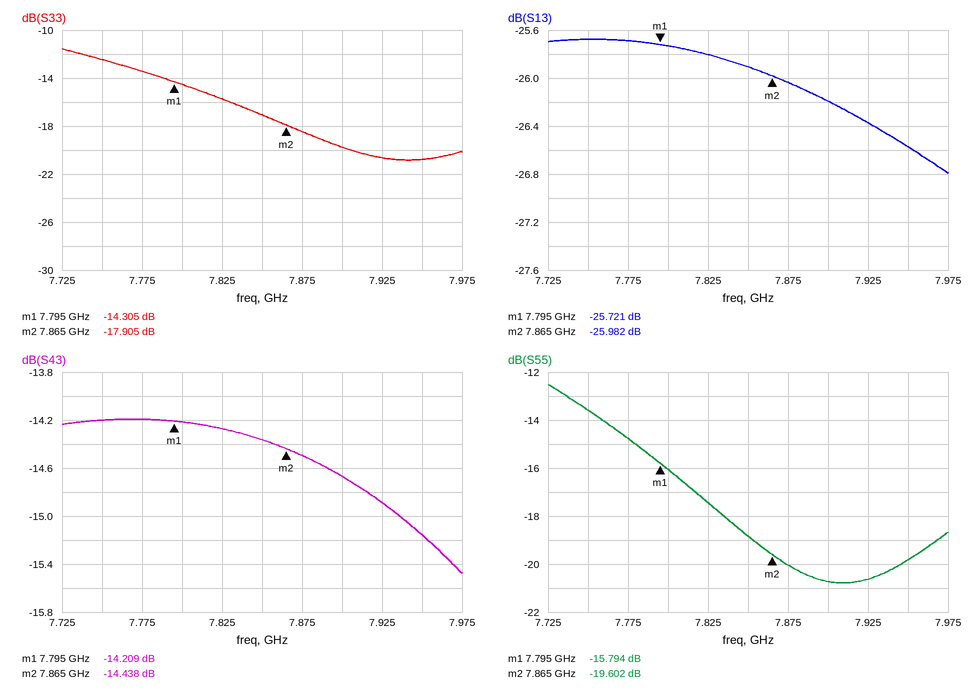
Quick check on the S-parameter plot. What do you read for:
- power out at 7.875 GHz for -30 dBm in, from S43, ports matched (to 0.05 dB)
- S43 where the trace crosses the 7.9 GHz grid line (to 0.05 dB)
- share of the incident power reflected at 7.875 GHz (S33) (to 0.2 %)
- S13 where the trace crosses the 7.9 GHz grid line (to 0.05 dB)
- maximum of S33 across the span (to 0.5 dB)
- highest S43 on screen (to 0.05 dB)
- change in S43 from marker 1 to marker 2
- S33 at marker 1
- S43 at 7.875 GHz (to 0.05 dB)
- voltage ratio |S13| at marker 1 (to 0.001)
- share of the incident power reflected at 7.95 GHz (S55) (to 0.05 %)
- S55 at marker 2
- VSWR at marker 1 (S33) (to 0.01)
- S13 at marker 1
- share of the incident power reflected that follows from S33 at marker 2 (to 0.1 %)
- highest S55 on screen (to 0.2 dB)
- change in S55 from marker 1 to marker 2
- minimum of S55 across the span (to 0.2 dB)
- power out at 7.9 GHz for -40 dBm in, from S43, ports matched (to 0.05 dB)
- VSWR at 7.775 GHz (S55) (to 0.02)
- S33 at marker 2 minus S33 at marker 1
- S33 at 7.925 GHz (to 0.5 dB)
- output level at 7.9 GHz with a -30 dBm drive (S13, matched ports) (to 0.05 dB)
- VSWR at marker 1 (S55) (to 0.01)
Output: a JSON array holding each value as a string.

["-44.50 dBm", "-14.65 dB", "1.4 %", "-26.20 dB", "-11.5 dB", "-14.20 dB", "-0.229 dB", "-14.305 dB", "-14.50 dB", "0.052", "1.05 %", "-19.602 dB", "1.48", "-25.721 dB", "1.6 %", "-12.6 dB", "-3.808 dB", "-20.8 dB", "-54.65 dBm", "1.44", "-3.600 dB", "-20.5 dB", "-56.20 dBm", "1.39"]
